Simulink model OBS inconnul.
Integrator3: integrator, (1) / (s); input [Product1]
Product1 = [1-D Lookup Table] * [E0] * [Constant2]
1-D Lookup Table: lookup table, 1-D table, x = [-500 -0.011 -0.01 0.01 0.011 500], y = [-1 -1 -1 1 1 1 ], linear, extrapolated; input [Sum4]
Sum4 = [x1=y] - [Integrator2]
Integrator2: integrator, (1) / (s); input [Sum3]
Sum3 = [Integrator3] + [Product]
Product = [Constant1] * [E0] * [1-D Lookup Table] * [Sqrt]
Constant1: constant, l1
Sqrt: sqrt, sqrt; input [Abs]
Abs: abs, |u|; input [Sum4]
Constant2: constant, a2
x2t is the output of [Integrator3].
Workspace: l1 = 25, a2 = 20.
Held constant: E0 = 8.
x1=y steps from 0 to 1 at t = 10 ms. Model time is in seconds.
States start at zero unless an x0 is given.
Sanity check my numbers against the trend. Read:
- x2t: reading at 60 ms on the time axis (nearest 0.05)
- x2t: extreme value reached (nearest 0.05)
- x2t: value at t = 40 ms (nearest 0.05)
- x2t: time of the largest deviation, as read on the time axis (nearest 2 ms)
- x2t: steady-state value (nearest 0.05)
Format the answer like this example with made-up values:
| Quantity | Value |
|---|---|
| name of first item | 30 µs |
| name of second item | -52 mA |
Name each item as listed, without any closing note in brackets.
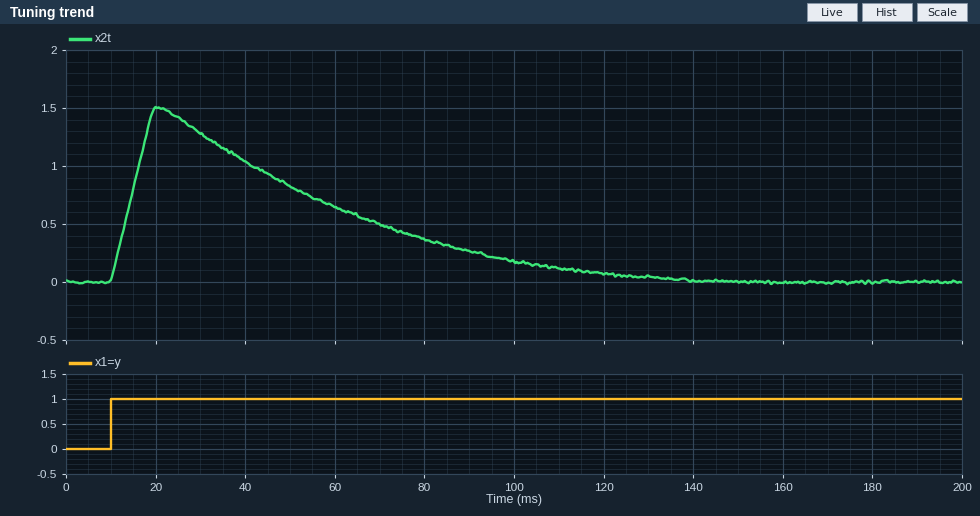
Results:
| Quantity | Value |
|---|---|
| x2t: reading at 60 ms on the time axis | 0.65 |
| x2t: extreme value reached | 1.50 |
| x2t: value at t = 40 ms | 1.05 |
| x2t: time of the largest deviation, as read on the time axis | 20 ms |
| x2t: steady-state value | 0.00 |
